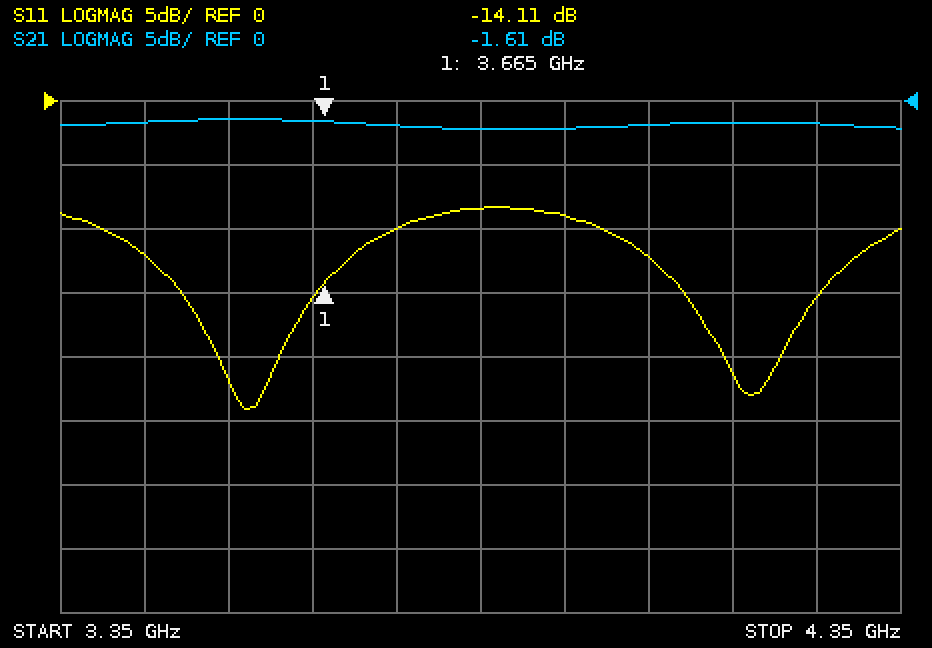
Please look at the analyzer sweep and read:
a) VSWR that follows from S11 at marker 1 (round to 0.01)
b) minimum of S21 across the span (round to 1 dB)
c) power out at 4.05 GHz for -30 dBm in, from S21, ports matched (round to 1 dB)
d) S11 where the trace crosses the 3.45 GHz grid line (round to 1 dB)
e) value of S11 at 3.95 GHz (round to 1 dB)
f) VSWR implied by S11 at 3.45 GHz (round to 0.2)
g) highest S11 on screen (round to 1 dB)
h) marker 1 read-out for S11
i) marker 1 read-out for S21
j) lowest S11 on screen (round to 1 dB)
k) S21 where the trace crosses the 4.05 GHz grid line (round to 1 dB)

1.49
-2 dB
-32 dBm
-12 dB
-9 dB
1.6
-8 dB
-14.11 dB
-1.61 dB
-24 dB
-2 dB
